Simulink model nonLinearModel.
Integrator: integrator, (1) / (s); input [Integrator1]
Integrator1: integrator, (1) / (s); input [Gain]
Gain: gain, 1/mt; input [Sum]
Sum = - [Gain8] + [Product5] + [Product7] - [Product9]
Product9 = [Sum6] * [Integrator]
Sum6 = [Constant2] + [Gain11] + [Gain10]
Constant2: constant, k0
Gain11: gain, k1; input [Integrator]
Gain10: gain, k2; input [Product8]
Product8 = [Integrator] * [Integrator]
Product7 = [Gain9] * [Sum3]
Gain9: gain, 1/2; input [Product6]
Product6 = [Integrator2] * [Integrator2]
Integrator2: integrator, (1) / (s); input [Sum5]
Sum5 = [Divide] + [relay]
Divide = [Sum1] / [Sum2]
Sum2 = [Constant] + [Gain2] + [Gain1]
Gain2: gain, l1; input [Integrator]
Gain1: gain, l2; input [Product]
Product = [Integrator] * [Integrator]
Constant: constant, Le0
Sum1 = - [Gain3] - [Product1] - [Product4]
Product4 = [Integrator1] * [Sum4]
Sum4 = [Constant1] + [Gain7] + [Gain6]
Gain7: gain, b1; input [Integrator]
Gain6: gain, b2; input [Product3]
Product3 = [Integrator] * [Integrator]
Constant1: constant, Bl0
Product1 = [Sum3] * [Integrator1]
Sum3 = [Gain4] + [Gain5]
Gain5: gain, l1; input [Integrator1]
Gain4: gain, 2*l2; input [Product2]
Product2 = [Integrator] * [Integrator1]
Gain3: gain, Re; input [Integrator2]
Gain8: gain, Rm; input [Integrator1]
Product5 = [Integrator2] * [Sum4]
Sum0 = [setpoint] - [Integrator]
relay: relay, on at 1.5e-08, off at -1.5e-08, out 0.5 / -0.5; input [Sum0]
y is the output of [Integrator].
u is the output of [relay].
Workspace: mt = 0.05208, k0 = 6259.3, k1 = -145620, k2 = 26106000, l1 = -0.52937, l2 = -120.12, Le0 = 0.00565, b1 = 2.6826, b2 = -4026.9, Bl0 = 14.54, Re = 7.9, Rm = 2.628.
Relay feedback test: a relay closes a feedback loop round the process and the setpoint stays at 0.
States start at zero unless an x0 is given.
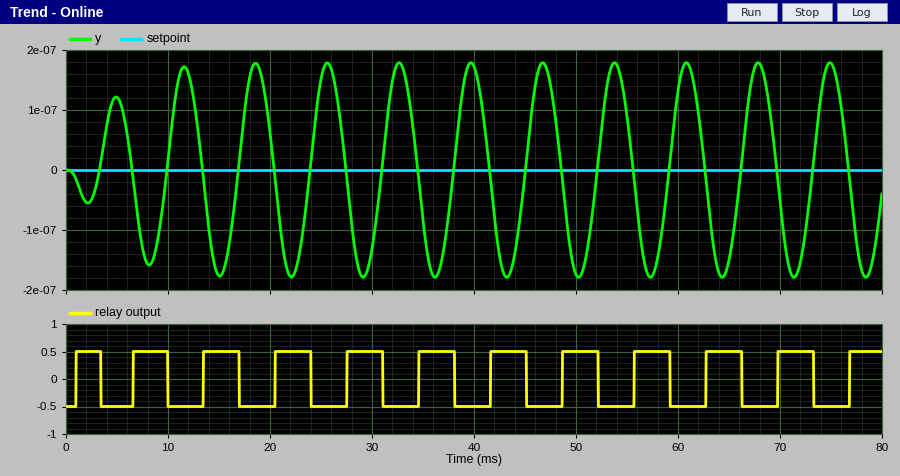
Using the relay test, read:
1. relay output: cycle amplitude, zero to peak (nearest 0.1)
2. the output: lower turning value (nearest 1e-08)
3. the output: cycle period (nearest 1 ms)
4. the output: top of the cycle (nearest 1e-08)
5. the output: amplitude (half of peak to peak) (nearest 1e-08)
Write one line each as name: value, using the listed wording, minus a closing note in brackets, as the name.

relay output: cycle amplitude, zero to peak: 0.5
the output: lower turning value: -0.00000018
the output: cycle period: 7 ms
the output: top of the cycle: 0.00000018
the output: amplitude (half of peak to peak): 0.00000018
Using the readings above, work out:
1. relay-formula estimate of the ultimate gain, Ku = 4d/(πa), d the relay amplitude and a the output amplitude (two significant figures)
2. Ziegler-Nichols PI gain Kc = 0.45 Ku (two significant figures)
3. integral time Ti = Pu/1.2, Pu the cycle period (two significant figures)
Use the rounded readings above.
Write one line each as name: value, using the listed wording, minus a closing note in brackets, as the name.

relay-formula estimate of the ultimate gain, Ku = 4d/(πa), d the relay amplitude and a the output amplitude: 3500000
Ziegler-Nichols PI gain Kc = 0.45 Ku: 1600000
integral time Ti = Pu/1.2, Pu the cycle period: 5.8 ms
